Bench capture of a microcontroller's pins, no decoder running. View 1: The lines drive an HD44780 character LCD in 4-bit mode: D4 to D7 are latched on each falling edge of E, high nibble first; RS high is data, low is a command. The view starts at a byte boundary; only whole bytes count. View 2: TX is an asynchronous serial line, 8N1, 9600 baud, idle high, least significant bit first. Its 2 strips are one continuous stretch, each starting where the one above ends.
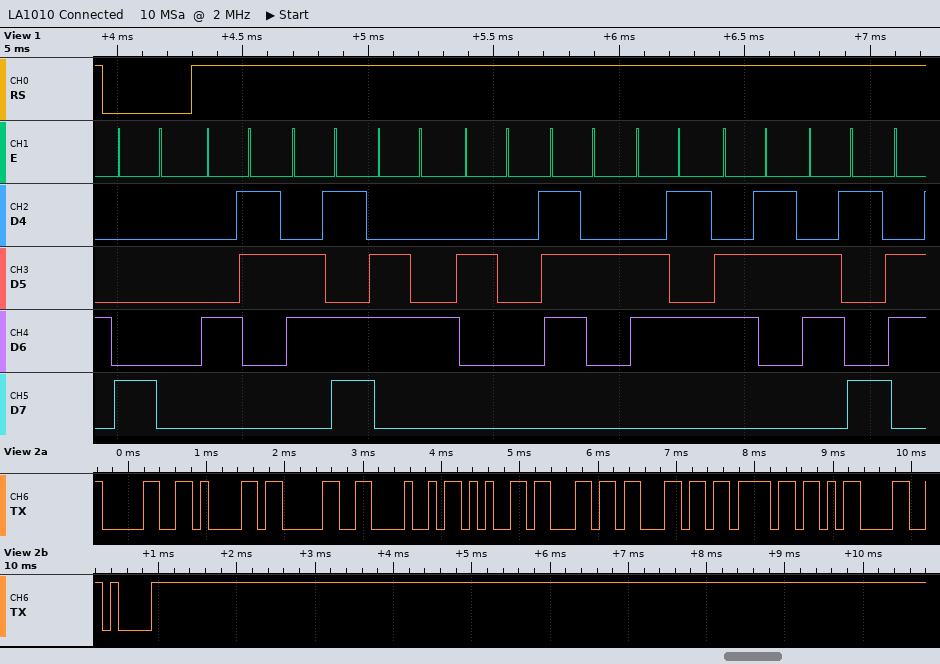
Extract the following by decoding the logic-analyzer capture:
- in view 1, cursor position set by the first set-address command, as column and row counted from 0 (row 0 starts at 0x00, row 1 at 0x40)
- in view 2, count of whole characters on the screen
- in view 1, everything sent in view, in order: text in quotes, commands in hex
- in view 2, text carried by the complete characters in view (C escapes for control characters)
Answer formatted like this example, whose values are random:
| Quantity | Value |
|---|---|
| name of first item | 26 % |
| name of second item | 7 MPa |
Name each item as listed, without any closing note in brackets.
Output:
| Quantity | Value |
|---|---|
| in view 1, cursor position set by the first set-address command, as column and row counted from 0 | column 0, row 0 |
| in view 2, count of whole characters on the screen | 10 |
| in view 1, everything sent in view, in order: text in quotes, commands in hex | 0x80 "Cmd reci" |
| in view 2, text carried by the complete characters in view | "0a0Hello\r\n" |
